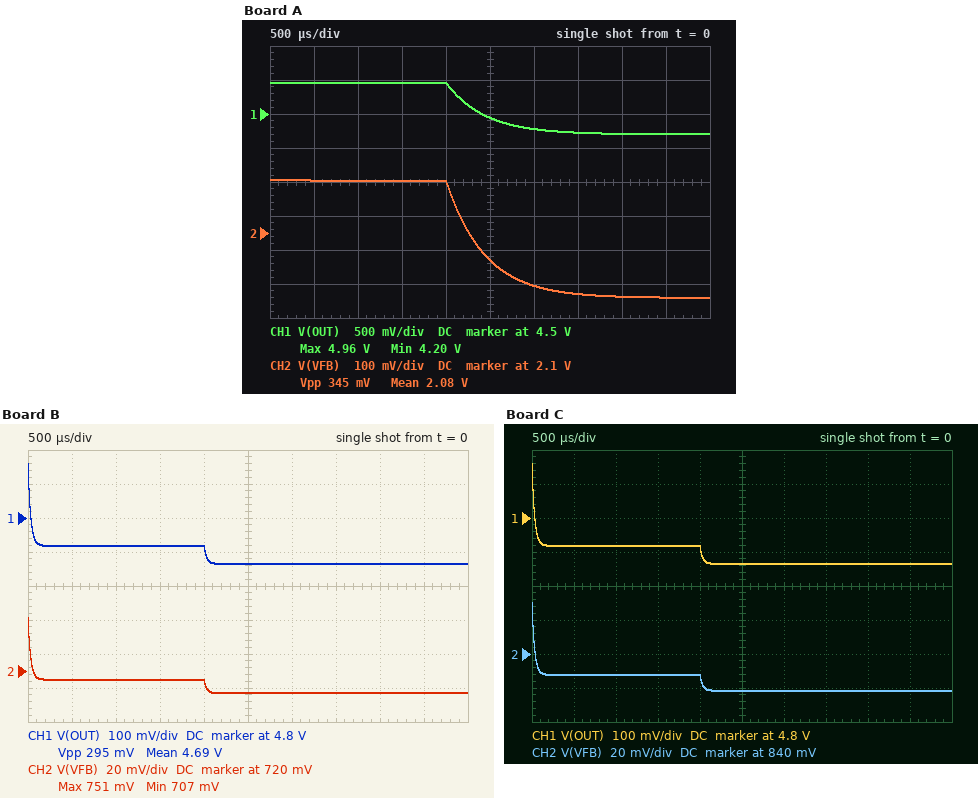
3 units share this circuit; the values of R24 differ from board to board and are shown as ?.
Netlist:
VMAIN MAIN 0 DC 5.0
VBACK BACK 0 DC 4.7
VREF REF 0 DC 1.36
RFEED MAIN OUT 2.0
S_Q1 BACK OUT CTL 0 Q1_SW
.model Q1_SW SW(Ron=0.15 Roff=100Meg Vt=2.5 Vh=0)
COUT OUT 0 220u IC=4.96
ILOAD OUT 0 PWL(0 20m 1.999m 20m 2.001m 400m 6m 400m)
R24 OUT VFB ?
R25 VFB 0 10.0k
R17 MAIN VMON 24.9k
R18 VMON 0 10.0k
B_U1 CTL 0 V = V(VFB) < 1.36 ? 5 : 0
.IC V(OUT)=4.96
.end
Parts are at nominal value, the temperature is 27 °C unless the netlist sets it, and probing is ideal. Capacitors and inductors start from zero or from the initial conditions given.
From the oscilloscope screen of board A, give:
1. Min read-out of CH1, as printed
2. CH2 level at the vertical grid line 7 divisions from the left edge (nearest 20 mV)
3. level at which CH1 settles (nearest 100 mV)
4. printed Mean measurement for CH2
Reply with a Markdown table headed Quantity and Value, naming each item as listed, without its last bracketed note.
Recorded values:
| Quantity | Value |
|---|---|
| Min read-out of CH1, as printed | 4.20 V |
| CH2 level at the vertical grid line 7 divisions from the left edge | 1.92 V |
| level at which CH1 settles | 4.2 V |
| printed Mean measurement for CH2 | 2.08 V |
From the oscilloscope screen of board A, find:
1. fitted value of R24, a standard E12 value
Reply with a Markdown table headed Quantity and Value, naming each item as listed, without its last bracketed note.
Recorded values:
| Quantity | Value |
|---|---|
| fitted value of R24, a standard E12 value | 12 kΩ |
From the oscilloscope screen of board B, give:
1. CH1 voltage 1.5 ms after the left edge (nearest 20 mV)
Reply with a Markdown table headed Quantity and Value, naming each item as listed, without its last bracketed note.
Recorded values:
| Quantity | Value |
|---|---|
| CH1 voltage 1.5 ms after the left edge | 4.72 V |
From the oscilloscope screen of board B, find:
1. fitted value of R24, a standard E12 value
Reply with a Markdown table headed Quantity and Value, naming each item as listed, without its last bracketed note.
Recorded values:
| Quantity | Value |
|---|---|
| fitted value of R24, a standard E12 value | 56 kΩ |
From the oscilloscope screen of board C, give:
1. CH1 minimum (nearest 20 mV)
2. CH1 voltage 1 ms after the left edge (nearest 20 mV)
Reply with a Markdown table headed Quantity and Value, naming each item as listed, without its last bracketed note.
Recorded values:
| Quantity | Value |
|---|---|
| CH1 minimum | 4.66 V |
| CH1 voltage 1 ms after the left edge | 4.72 V |
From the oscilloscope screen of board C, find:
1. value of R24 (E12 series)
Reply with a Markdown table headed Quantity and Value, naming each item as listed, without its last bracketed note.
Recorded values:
| Quantity | Value |
|---|---|
| value of R24 | 47 kΩ |
